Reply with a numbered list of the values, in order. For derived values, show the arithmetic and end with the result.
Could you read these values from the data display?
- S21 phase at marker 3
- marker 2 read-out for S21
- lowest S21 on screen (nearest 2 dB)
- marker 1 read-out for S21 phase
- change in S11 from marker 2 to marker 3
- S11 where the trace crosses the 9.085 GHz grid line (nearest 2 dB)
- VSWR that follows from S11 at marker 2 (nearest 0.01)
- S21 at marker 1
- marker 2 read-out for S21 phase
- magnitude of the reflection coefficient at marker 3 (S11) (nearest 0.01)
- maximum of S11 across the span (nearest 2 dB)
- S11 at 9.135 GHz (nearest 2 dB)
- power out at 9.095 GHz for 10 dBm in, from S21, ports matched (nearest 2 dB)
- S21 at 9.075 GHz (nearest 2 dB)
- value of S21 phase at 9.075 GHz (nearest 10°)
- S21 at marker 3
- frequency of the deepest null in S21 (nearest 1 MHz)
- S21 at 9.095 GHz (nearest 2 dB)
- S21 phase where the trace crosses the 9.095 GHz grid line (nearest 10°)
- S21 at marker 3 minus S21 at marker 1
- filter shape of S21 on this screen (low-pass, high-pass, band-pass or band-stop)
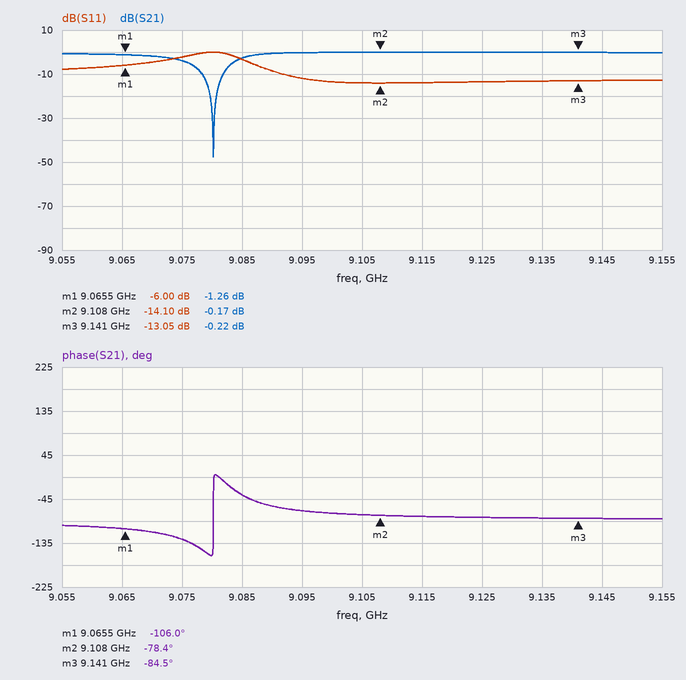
1. -84.5°
2. -0.17 dB
3. -48 dB
4. -106.0°
5. -13.05 − (-14.1) = 1.05 dB
6. -4 dB
7. (1 + 0.1972)/(1 − 0.1972) ≈ 1.49
8. -1.26 dB
9. -78.4°
10. 10^(-13.05/20) ≈ 0.22
11. 0 dB
12. -14 dB
13. 10 dBm + (0 dB) = 10 dBm
14. -4 dB
15. -130°
16. -0.22 dB
17. 9.080 GHz
18. 0 dB
19. -70°
20. -0.22 − (-1.26) = 1.04 dB
21. band-stop
